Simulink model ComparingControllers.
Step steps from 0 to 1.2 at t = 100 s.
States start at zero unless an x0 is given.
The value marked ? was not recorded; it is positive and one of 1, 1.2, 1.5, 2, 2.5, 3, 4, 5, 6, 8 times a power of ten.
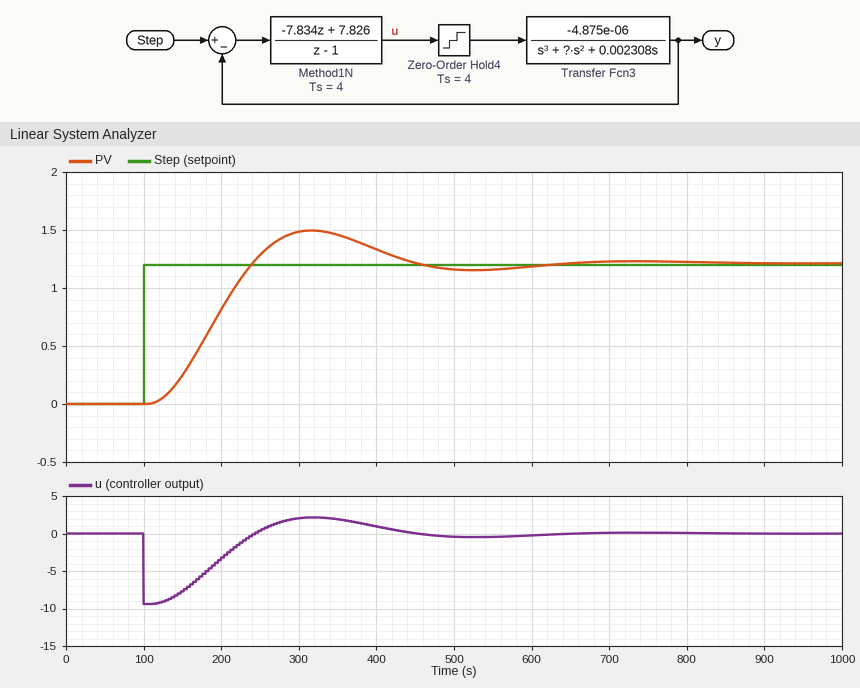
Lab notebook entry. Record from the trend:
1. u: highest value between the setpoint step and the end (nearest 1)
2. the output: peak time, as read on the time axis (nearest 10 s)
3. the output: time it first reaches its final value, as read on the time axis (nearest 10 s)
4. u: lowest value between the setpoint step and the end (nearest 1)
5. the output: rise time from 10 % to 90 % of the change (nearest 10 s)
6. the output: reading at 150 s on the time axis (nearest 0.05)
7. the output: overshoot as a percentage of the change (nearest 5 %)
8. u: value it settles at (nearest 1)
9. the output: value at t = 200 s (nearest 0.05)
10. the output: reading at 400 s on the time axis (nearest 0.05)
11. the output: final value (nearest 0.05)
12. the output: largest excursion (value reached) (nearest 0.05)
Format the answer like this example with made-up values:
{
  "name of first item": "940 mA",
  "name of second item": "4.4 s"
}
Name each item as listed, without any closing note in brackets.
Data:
{
  "u: highest value between the setpoint step and the end": "2",
  "the output: peak time, as read on the time axis": "320 s",
  "the output: time it first reaches its final value, as read on the time axis": "240 s",
  "u: lowest value between the setpoint step and the end": "-9",
  "the output: rise time from 10 % to 90 % of the change": "90 s",
  "the output: reading at 150 s on the time axis": "0.25",
  "the output: overshoot as a percentage of the change": "25 %",
  "u: value it settles at": "0",
  "the output: value at t = 200 s": "0.80",
  "the output: reading at 400 s on the time axis": "1.35",
  "the output: final value": "1.20",
  "the output: largest excursion (value reached)": "1.50"
}
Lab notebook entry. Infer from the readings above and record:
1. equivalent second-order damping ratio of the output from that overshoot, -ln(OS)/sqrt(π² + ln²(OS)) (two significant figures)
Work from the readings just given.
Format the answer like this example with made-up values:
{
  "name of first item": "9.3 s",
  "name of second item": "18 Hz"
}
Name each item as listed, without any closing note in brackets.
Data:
{
  "equivalent second-order damping ratio of the output from that overshoot, -ln(OS)/sqrt(π² + ln²(OS))": "0.40"
}
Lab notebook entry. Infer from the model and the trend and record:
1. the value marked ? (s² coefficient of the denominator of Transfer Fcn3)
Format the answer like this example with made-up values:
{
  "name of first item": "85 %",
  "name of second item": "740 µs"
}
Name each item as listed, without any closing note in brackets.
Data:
{
  "the value marked ?": "0.15"
}
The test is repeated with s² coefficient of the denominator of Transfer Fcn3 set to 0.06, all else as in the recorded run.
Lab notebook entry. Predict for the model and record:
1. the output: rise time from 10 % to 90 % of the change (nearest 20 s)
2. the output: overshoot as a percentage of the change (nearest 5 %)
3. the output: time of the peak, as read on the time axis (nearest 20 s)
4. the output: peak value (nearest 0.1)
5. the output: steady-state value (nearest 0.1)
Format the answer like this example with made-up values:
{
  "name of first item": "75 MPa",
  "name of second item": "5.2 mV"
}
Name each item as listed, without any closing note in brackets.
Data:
{
  "the output: rise time from 10 % to 90 % of the change": "60 s",
  "the output: overshoot as a percentage of the change": "10 %",
  "the output: time of the peak, as read on the time axis": "240 s",
  "the output: peak value": "1.3",
  "the output: steady-state value": "1.2"
}
